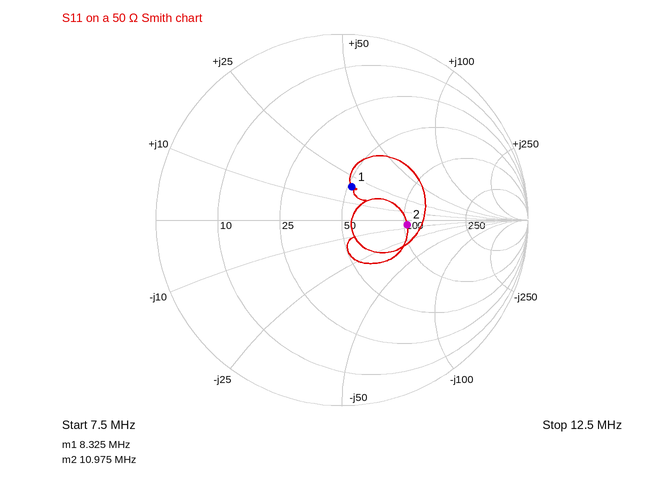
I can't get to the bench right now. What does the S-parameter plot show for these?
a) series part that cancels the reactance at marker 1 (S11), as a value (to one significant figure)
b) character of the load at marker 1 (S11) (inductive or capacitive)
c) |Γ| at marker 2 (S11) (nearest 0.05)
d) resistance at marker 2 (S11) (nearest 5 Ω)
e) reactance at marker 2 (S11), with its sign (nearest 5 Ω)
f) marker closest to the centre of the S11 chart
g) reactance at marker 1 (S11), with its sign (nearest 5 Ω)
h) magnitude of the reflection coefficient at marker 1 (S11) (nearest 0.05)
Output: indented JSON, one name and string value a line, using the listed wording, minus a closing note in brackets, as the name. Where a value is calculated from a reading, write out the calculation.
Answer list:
{
  "series part that cancels the reactance at marker 1 (S11), as a value": "C = 1/(2π × 8.325 MHz × 20 Ω) ≈ 1.0 nF",
  "character of the load at marker 1 (S11)": "inductive",
  "|Γ| at marker 2 (S11)": "0.35",
  "resistance at marker 2 (S11)": "105 Ω",
  "reactance at marker 2 (S11), with its sign": "-5 Ω",
  "marker closest to the centre of the S11 chart": "marker 1",
  "reactance at marker 1 (S11), with its sign": "+20 Ω",
  "magnitude of the reflection coefficient at marker 1 (S11)": "0.20"
}
